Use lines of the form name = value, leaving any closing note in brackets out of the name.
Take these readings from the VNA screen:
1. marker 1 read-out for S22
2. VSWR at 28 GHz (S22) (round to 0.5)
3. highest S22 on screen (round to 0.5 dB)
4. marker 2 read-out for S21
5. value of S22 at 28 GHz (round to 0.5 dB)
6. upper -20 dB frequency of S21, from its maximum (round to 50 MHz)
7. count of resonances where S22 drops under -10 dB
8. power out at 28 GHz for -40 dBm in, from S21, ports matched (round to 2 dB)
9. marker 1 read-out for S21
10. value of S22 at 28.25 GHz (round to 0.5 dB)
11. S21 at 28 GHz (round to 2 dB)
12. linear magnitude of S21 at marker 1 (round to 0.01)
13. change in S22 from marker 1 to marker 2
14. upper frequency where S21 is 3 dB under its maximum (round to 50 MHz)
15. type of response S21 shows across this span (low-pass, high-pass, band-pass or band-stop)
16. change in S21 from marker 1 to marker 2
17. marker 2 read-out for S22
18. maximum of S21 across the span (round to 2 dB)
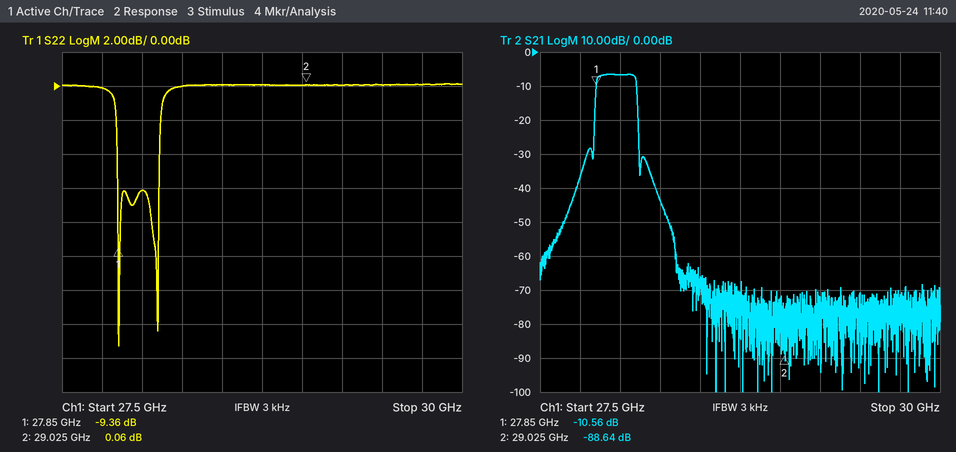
marker 1 read-out for S22 = -9.36 dB
VSWR at 28 GHz (S22) = 3.0
highest S22 on screen = 0.0 dB
marker 2 read-out for S21 = -88.64 dB
value of S22 at 28 GHz = -6.0 dB
upper -20 dB frequency of S21, from its maximum = 28.10 GHz
count of resonances where S22 drops under -10 dB = 2
power out at 28 GHz for -40 dBm in, from S21, ports matched = -46 dBm
marker 1 read-out for S21 = -10.56 dB
value of S22 at 28.25 GHz = 0.0 dB
S21 at 28 GHz = -6 dB
linear magnitude of S21 at marker 1 = 0.30
change in S22 from marker 1 to marker 2 = 9.42 dB
upper frequency where S21 is 3 dB under its maximum = 28.10 GHz
type of response S21 shows across this span = band-pass
change in S21 from marker 1 to marker 2 = -78.08 dB
marker 2 read-out for S22 = 0.06 dB
maximum of S21 across the span = -6 dB
